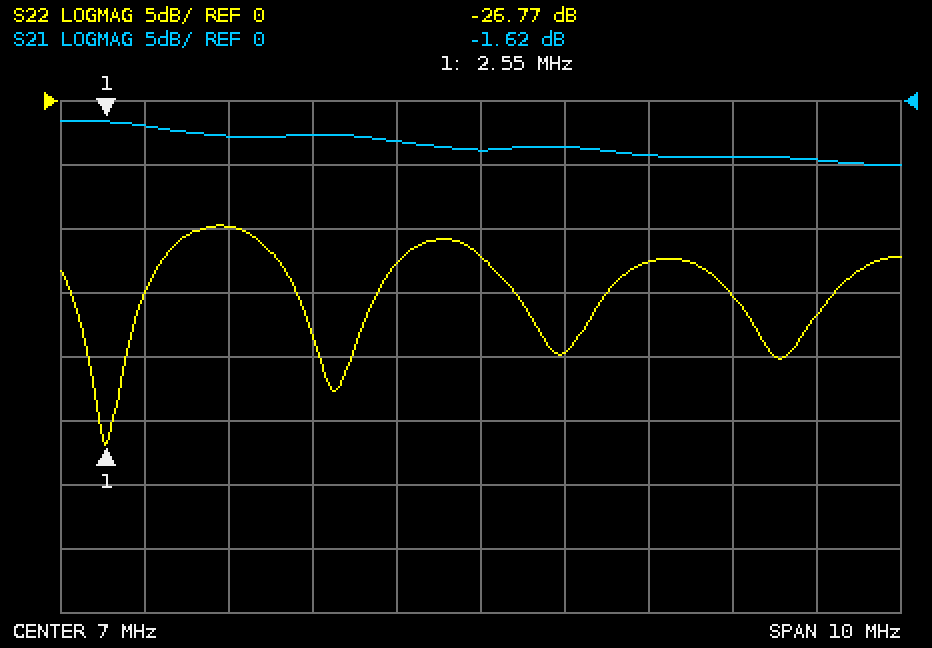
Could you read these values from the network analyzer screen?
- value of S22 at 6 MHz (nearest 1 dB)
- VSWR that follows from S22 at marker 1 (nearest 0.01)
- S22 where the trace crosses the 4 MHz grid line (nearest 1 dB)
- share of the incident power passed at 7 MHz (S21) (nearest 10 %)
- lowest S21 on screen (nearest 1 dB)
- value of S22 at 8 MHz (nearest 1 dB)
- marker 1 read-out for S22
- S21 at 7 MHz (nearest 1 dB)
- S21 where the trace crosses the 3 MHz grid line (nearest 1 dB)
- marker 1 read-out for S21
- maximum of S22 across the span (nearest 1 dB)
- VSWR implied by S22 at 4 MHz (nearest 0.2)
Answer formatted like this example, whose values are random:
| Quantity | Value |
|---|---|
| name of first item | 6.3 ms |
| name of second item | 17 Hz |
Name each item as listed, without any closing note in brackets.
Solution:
| Quantity | Value |
|---|---|
| value of S22 at 6 MHz | -13 dB |
| VSWR that follows from S22 at marker 1 | 1.10 |
| S22 where the trace crosses the 4 MHz grid line | -10 dB |
| share of the incident power passed at 7 MHz (S21) | 40 % |
| lowest S21 on screen | -5 dB |
| value of S22 at 8 MHz | -20 dB |
| marker 1 read-out for S22 | -26.77 dB |
| S21 at 7 MHz | -4 dB |
| S21 where the trace crosses the 3 MHz grid line | -2 dB |
| marker 1 read-out for S21 | -1.62 dB |
| maximum of S22 across the span | -10 dB |
| VSWR implied by S22 at 4 MHz | 2.0 |
